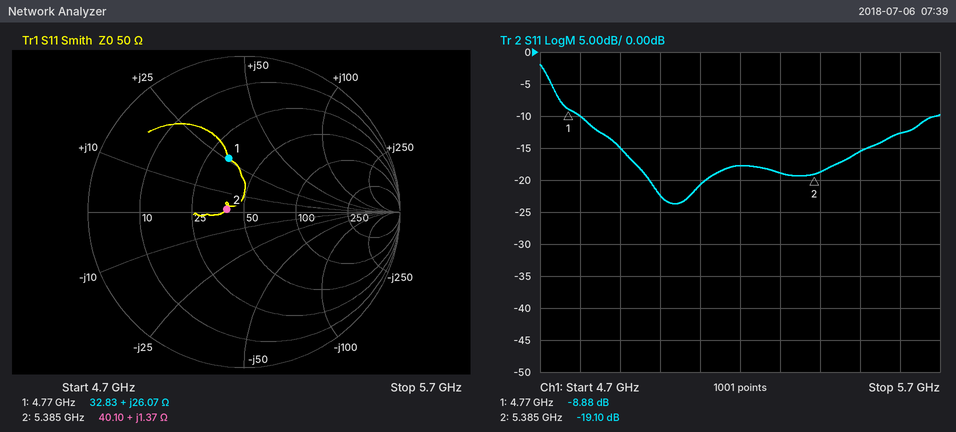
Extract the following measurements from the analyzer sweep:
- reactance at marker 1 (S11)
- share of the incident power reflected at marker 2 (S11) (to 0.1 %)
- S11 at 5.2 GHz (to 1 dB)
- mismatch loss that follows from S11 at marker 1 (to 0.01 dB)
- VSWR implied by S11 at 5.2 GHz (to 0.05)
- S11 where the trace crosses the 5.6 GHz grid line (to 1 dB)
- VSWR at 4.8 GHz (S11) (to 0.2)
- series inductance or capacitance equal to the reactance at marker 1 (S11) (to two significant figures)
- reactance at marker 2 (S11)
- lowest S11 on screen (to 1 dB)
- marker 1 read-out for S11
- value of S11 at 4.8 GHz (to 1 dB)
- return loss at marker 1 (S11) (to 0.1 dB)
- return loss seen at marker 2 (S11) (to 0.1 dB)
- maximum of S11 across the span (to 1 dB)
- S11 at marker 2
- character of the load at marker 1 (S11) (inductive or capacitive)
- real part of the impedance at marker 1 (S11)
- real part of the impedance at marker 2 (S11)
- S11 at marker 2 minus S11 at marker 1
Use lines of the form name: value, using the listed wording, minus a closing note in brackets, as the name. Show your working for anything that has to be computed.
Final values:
reactance at marker 1: +26.07 Ω
share of the incident power reflected at marker 2 (S11): 10^(-19.1/10) ≈ 1.2 %
S11 at 5.2 GHz: -18 dB
mismatch loss that follows from S11 at marker 1: −10 log10(1 − 10^(-8.88/10)) ≈ 0.60 dB
VSWR implied by S11 at 5.2 GHz: |Γ| = 10^(-18/20) = 0.1259; VSWR = (1 + 0.1259)/(1 − 0.1259) ≈ 1.29, so 1.30 to the nearest 0.05
S11 where the trace crosses the 5.6 GHz grid line: -13 dB
VSWR at 4.8 GHz (S11): |Γ| = 10^(-10/20) = 0.3162; VSWR = (1 + 0.3162)/(1 − 0.3162) ≈ 1.92, so 2.0 to the nearest 0.2
series inductance or capacitance equal to the reactance at marker 1 (S11): L = 26.07 Ω/(2π × 4.77 GHz) ≈ 870 pH
reactance at marker 2: +1.37 Ω
lowest S11 on screen: -24 dB
marker 1 read-out for S11: -8.88 dB
value of S11 at 4.8 GHz: -10 dB
return loss at marker 1 (S11): 8.9 dB
return loss seen at marker 2 (S11): 19.1 dB
maximum of S11 across the span: -2 dB
S11 at marker 2: -19.10 dB
character of the load at marker 1 (S11): inductive
real part of the impedance at marker 1: 32.83 Ω
real part of the impedance at marker 2: 40.10 Ω
S11 at marker 2 minus S11 at marker 1: -19.1 − (-8.88) = -10.22 dB
